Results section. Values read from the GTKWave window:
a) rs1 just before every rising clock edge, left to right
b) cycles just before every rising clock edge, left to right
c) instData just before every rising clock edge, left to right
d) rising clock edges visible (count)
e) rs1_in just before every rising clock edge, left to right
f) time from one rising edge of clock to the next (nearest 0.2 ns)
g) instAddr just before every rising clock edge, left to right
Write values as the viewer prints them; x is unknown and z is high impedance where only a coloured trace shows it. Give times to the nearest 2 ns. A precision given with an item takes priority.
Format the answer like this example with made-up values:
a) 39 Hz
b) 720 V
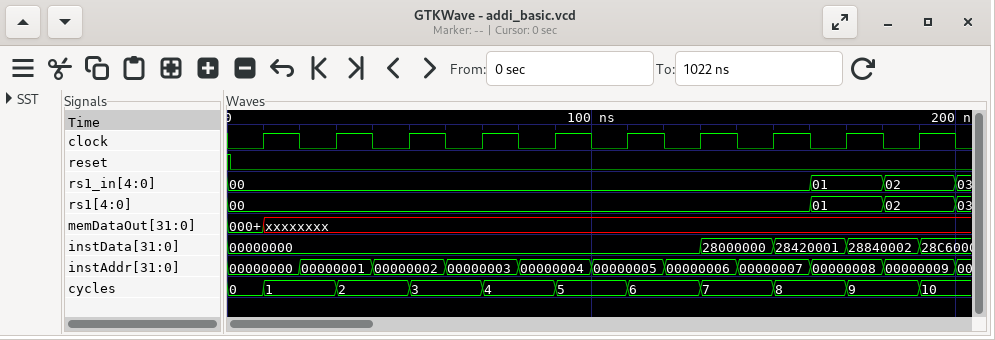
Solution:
a) 00, 00, 00, 00, 00, 00, 00, 00, 01, 02
b) 0, 1, 2, 3, 4, 5, 6, 7, 8, 9
c) 00000000, 00000000, 00000000, 00000000, 00000000, 00000000, 00000000, 28000000, 28420001, 28840002
d) 10
e) 00, 00, 00, 00, 00, 00, 00, 00, 01, 02
f) 20 ns
g) 00000000, 00000001, 00000002, 00000003, 00000004, 00000005, 00000006, 00000007, 00000008, 00000009
